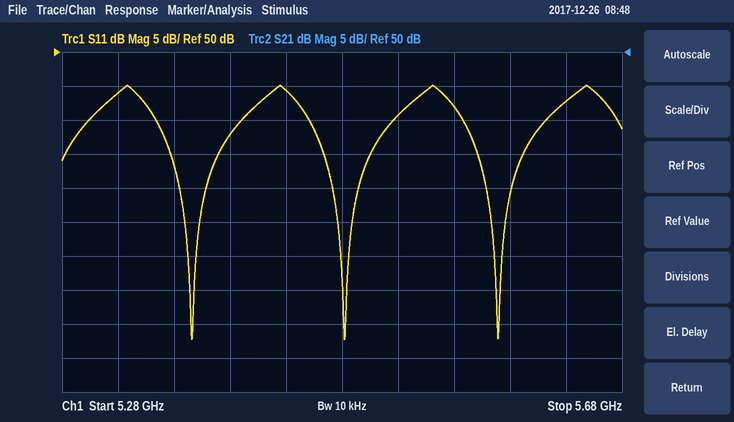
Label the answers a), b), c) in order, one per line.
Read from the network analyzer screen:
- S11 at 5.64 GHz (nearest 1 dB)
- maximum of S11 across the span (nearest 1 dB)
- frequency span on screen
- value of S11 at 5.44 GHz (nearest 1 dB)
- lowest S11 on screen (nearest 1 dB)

a) 43 dB
b) 45 dB
c) 400 MHz
d) 44 dB
e) 8 dB
